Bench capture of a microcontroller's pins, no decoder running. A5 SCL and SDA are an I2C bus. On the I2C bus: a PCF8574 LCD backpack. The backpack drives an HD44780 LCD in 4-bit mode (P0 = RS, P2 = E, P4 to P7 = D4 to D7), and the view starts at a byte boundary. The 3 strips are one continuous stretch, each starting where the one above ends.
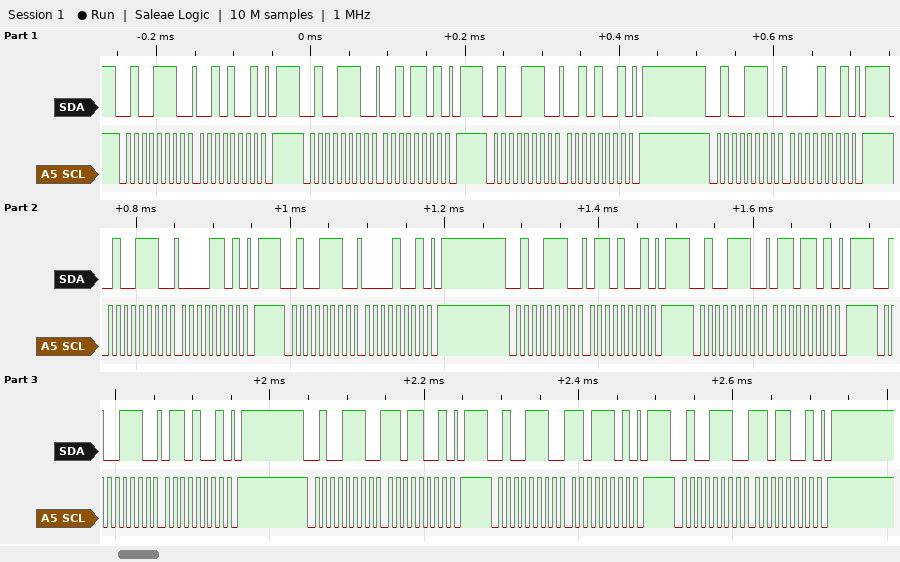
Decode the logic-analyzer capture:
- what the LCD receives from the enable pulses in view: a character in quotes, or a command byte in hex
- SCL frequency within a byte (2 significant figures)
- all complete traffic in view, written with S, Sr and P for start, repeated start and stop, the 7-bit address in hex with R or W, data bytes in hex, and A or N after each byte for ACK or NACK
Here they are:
' ' 'm'
100 kHz
S 27W A 29 A P S 27W A 2D A P S 27W A 29 A P S 27W A 09 A P S 27W A 0D A P S 27W A 09 A P S 27W A 69 A P S 27W A 6D A P S 27W A 69 A P S 27W A D9 A P S 27W A DD A P S 27W A D9 A P
